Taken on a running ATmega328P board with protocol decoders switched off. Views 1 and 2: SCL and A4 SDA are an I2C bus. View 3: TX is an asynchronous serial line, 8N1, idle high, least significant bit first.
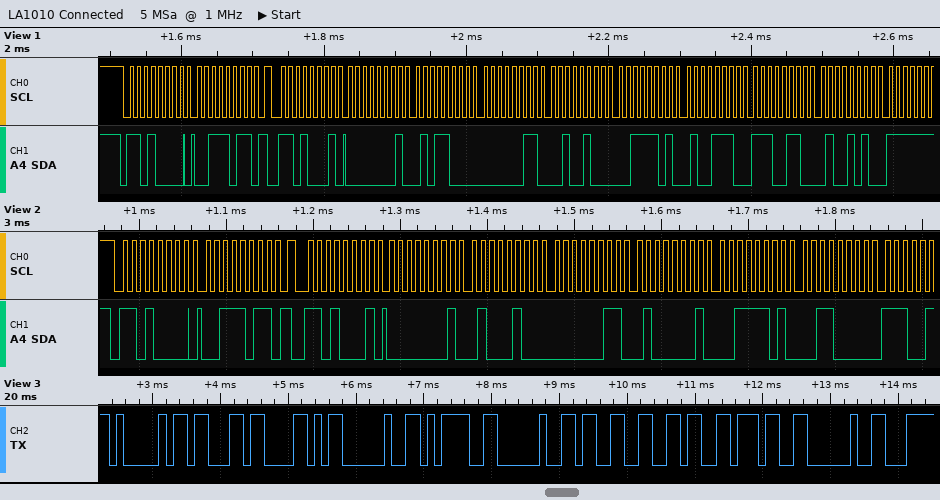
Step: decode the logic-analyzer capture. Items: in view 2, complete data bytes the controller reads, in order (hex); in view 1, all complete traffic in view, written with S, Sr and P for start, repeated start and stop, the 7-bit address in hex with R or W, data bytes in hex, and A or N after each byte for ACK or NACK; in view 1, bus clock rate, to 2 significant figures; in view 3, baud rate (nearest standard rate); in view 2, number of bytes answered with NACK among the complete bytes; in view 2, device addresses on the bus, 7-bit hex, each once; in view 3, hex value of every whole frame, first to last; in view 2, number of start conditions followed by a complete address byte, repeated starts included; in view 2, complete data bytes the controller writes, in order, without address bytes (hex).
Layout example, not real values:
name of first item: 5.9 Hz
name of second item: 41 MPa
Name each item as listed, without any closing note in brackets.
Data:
in view 2, complete data bytes the controller reads, in order: 01 44 03 41 3D 30
in view 1, all complete traffic in view, written with S, Sr and P for start, repeated start and stop, the 7-bit address in hex with R or W, data bytes in hex, and A or N after each byte for ACK or NACK: S 68W A 3B A Sr 68R A 01 A 58 A 03 A 24 A 3D A 4E A E6 A 4A A
in view 1, bus clock rate, to 2 significant figures: 100 kHz
in view 3, baud rate: 9600 baud
in view 2, number of bytes answered with NACK among the complete bytes: 0
in view 2, device addresses on the bus, 7-bit hex, each once: 0x68
in view 3, hex value of every whole frame, first to last: 41 63 58 20 3D 20 33 36 37 20
in view 2, number of start conditions followed by a complete address byte, repeated starts included: 2
in view 2, complete data bytes the controller writes, in order, without address bytes: 3B
